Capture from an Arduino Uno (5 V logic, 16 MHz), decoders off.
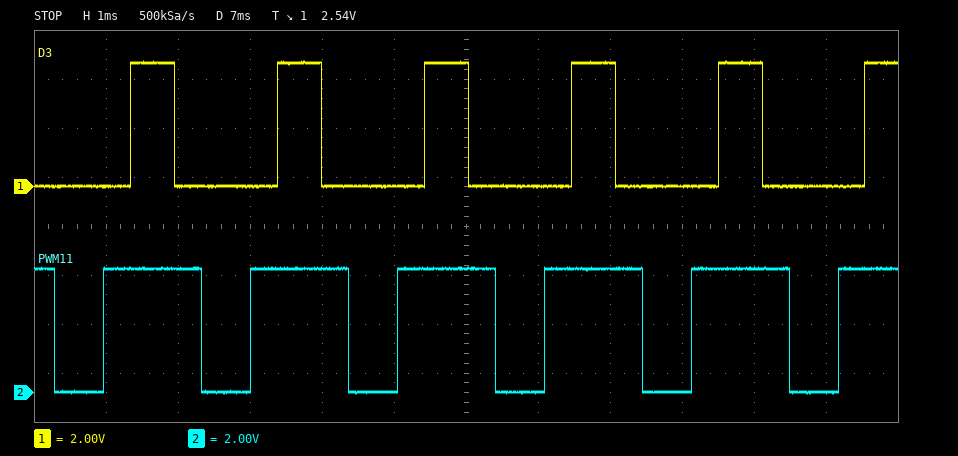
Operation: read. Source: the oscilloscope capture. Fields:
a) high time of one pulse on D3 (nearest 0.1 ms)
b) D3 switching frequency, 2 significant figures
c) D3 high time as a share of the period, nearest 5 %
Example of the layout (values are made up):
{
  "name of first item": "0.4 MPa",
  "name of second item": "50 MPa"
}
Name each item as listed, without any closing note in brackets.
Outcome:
{
  "high time of one pulse on D3": "0.6 ms",
  "D3 switching frequency, 2 significant figures": "490 Hz",
  "D3 high time as a share of the period, nearest 5 %": "30 %"
}
